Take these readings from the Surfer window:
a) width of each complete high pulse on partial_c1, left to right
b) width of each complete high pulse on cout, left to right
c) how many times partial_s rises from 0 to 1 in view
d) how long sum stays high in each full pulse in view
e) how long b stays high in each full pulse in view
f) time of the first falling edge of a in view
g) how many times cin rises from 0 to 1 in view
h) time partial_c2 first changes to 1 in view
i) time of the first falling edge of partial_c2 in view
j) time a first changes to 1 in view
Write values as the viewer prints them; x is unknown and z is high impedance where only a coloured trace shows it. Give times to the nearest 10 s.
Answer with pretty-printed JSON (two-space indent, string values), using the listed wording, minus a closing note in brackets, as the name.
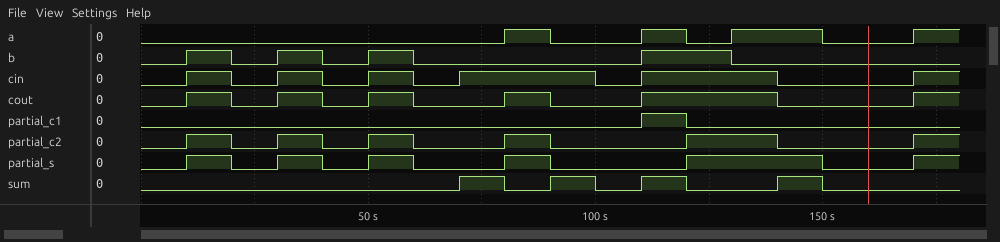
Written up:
{
  "width of each complete high pulse on partial_c1, left to right": "10 s",
  "width of each complete high pulse on cout, left to right": "10 s, 10 s, 10 s, 10 s, 30 s",
  "how many times partial_s rises from 0 to 1 in view": "6",
  "how long sum stays high in each full pulse in view": "10 s, 10 s, 10 s, 10 s",
  "how long b stays high in each full pulse in view": "10 s, 10 s, 10 s, 20 s",
  "time of the first falling edge of a in view": "90 s",
  "how many times cin rises from 0 to 1 in view": "6",
  "time partial_c2 first changes to 1 in view": "10 s",
  "time of the first falling edge of partial_c2 in view": "20 s",
  "time a first changes to 1 in view": "80 s"
}
